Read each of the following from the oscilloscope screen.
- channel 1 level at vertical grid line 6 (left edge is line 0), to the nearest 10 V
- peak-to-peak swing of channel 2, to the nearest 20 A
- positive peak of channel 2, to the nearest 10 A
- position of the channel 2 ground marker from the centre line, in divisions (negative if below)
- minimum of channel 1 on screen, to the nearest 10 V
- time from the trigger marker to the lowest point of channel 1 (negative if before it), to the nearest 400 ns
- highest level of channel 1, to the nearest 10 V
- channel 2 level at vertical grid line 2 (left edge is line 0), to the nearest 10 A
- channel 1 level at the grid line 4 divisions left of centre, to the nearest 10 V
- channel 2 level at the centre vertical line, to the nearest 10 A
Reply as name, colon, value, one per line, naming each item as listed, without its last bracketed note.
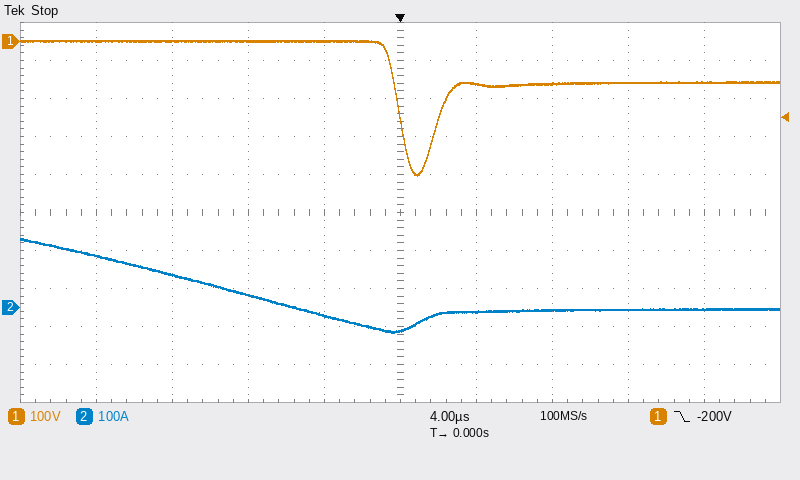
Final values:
channel 1 level at vertical grid line 6 (left edge is line 0), to the nearest 10 V: -110 V
peak-to-peak swing of channel 2, to the nearest 20 A: 240 A
positive peak of channel 2, to the nearest 10 A: 180 A
position of the channel 2 ground marker from the centre line, in divisions: -2.5 div
minimum of channel 1 on screen, to the nearest 10 V: -350 V
time from the trigger marker to the lowest point of channel 1 (negative if before it), to the nearest 400 ns: +800 ns
highest level of channel 1, to the nearest 10 V: 0 V
channel 2 level at vertical grid line 2 (left edge is line 0), to the nearest 10 A: 90 A
channel 1 level at the grid line 4 divisions left of centre, to the nearest 10 V: 0 V
channel 2 level at the centre vertical line, to the nearest 10 A: -60 A
